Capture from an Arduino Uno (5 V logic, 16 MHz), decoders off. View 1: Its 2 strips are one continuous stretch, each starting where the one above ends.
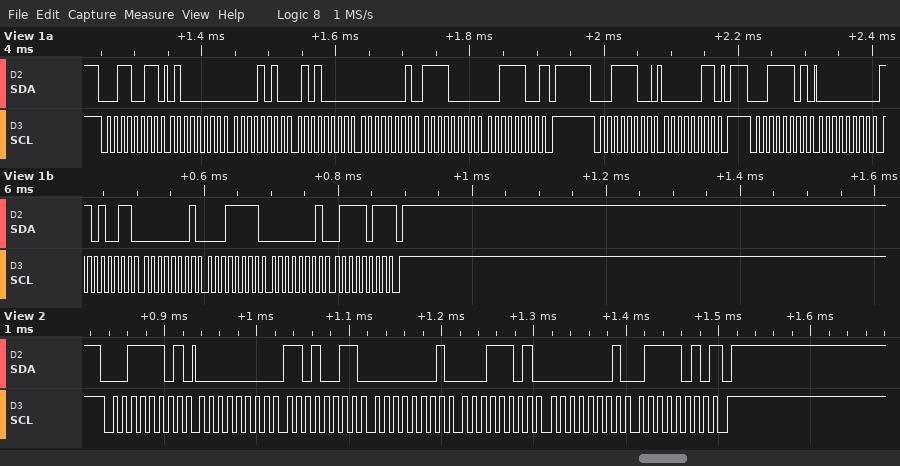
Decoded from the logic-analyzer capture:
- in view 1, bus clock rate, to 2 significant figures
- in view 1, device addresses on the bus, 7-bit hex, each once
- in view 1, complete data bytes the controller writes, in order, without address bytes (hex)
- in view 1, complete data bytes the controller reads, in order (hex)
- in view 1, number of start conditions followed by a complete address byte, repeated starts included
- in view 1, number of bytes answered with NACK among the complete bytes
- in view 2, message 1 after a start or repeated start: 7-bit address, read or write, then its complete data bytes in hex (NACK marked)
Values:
100 kHz
0x19 0x1E
03
40 0A 50 01 F0 3C 00 D3 01 1F 01 7B
3
2
0x1E read: 00 D3 01 1D 01 7A NACK
